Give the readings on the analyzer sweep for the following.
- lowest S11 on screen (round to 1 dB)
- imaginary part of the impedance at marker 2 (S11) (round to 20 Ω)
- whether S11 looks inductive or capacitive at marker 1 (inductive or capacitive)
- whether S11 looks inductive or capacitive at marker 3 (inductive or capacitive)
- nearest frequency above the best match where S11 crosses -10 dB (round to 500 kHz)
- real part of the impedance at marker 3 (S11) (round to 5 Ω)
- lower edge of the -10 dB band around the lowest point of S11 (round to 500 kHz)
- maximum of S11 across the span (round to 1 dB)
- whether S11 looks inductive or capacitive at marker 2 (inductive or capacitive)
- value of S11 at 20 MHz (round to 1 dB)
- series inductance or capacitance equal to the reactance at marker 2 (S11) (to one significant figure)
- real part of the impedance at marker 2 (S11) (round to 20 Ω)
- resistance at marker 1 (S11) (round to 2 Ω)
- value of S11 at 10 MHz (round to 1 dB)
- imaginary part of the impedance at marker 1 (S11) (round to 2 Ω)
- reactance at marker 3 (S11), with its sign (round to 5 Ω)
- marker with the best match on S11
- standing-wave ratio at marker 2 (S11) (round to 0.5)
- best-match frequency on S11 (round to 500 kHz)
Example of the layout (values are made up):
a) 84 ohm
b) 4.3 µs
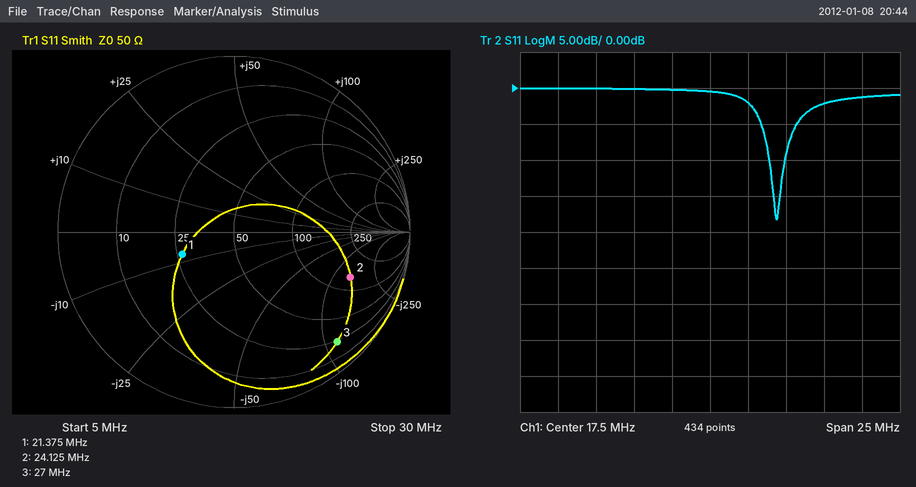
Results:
a) -18 dB
b) -140 Ω
c) capacitive
d) capacitive
e) 22.5 MHz
f) 25 Ω
g) 21.5 MHz
h) 0 dB
i) capacitive
j) -2 dB
k) 50 pF
l) 140 Ω
m) 26 Ω
n) 0 dB
o) -8 Ω
p) -110 Ω
q) marker 1
r) 6.0
s) 22.0 MHz
